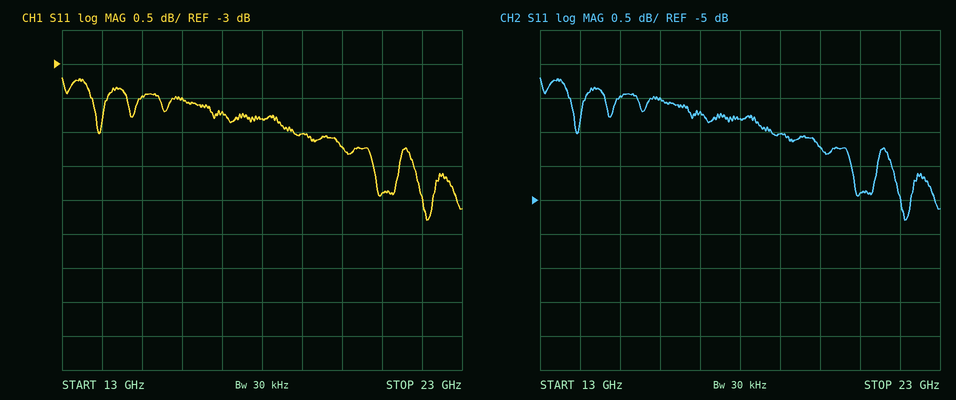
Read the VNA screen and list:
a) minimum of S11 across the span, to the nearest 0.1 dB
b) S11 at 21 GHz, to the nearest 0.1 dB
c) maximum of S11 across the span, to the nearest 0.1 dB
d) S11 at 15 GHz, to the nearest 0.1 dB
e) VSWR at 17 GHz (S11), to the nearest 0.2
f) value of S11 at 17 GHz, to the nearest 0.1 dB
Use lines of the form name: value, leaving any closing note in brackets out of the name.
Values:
minimum of S11 across the span, to the nearest 0.1 dB: -5.3 dB
S11 at 21 GHz, to the nearest 0.1 dB: -4.9 dB
maximum of S11 across the span, to the nearest 0.1 dB: -3.2 dB
S11 at 15 GHz, to the nearest 0.1 dB: -3.5 dB
VSWR at 17 GHz (S11), to the nearest 0.2: 4.8
value of S11 at 17 GHz, to the nearest 0.1 dB: -3.7 dB
